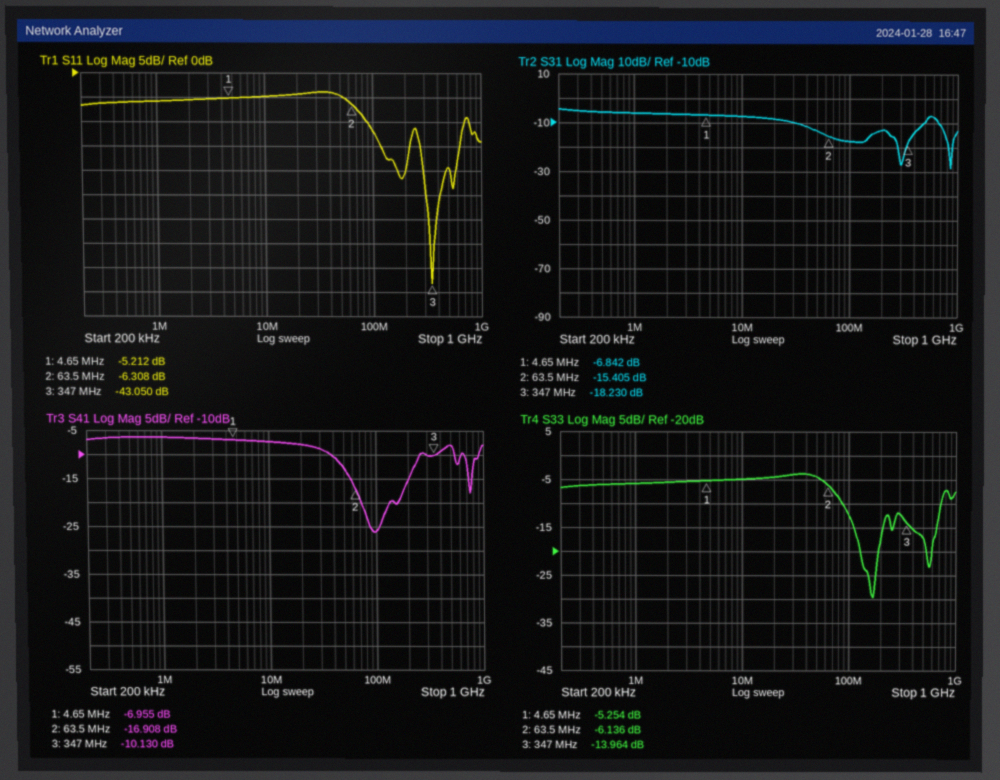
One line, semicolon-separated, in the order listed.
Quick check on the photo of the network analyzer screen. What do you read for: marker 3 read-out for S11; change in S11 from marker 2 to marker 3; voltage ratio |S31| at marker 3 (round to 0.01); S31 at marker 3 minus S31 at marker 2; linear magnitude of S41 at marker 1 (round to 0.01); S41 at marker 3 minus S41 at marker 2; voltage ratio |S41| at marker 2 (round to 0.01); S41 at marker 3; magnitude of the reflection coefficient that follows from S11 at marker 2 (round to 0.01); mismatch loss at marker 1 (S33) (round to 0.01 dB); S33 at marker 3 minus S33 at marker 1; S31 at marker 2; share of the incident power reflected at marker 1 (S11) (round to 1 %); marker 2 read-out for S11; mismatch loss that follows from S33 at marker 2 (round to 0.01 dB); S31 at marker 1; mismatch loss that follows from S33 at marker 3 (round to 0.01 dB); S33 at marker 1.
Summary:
-43.050 dB; -36.742 dB; 0.12; -2.825 dB; 0.45; 6.778 dB; 0.14; -10.130 dB; 0.48; 1.54 dB; -8.710 dB; -15.405 dB; 30 %; -6.308 dB; 1.21 dB; -6.842 dB; 0.18 dB; -5.254 dB
